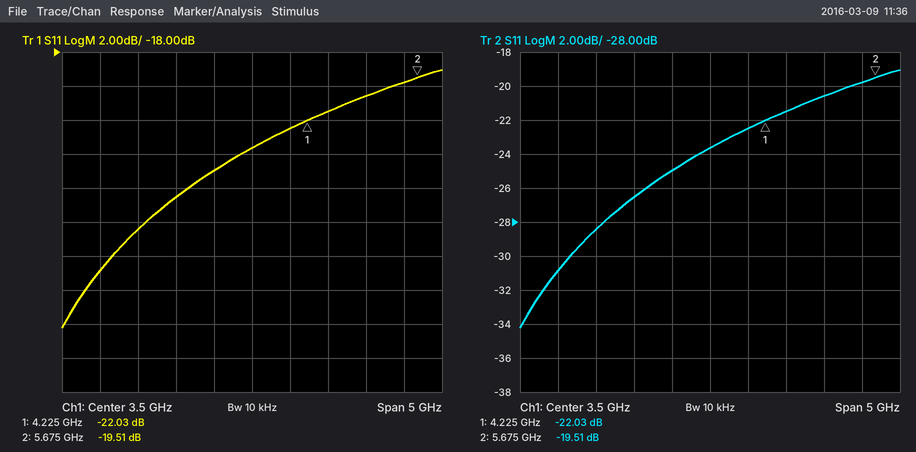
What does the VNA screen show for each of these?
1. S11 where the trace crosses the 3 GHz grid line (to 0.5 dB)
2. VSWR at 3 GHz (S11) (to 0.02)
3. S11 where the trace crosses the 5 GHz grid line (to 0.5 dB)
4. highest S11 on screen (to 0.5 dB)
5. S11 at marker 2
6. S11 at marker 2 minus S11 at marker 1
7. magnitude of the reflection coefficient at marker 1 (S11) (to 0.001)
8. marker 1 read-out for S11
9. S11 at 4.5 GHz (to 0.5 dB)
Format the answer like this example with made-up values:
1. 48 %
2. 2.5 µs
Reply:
1. -25.0 dB
2. 1.12
3. -20.5 dB
4. -19.0 dB
5. -19.51 dB
6. 2.52 dB
7. 0.079
8. -22.03 dB
9. -21.5 dB
